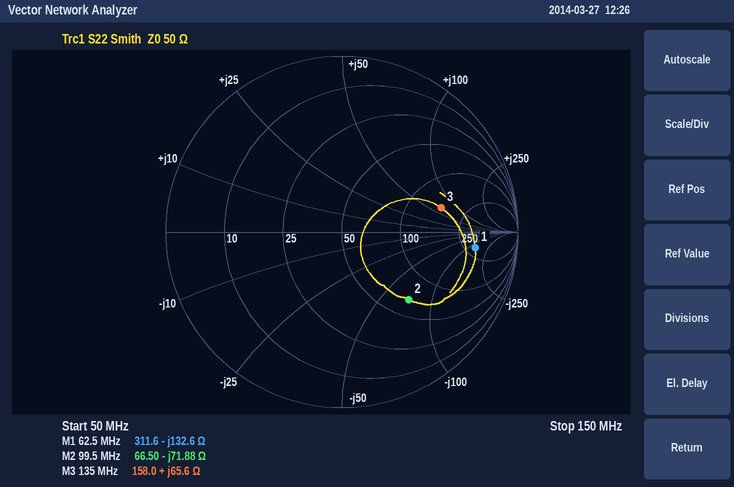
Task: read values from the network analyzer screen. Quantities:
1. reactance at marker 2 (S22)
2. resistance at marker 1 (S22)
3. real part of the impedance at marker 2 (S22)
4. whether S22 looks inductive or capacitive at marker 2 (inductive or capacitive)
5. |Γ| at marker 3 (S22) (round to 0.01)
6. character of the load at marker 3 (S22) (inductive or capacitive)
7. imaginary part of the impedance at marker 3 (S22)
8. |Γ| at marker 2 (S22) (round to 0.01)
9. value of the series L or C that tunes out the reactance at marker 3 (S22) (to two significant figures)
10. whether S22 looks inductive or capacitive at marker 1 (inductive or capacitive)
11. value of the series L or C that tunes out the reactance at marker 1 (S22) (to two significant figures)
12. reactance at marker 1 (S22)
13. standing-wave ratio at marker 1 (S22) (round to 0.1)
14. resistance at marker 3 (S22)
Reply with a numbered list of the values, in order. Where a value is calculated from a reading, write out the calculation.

1. -71.88 Ω
2. 311.6 Ω
3. 66.50 Ω
4. capacitive
5. 0.58
6. inductive
7. +65.6 Ω
8. 0.54
9. C = 1/(2π × 135 MHz × 65.6 Ω) ≈ 18 pF
10. capacitive
11. L = 132.6 Ω/(2π × 62.5 MHz) ≈ 338 nH, so 340 nH to two significant figures
12. -132.6 Ω
13. 7.4
14. 158.0 Ω
